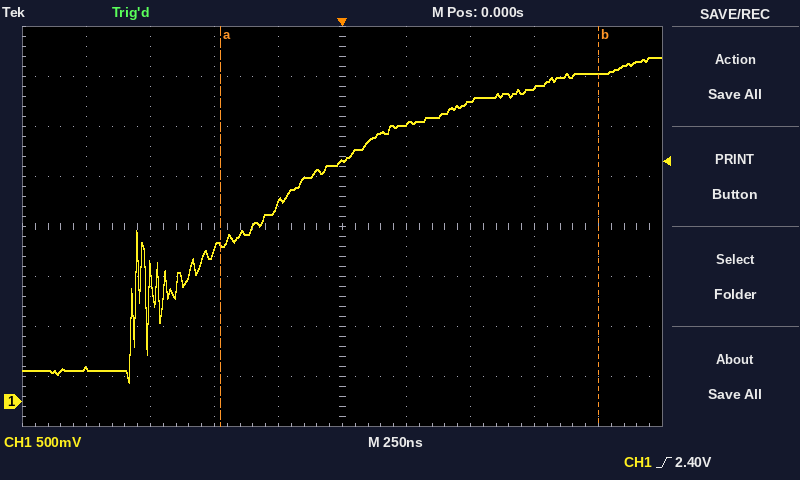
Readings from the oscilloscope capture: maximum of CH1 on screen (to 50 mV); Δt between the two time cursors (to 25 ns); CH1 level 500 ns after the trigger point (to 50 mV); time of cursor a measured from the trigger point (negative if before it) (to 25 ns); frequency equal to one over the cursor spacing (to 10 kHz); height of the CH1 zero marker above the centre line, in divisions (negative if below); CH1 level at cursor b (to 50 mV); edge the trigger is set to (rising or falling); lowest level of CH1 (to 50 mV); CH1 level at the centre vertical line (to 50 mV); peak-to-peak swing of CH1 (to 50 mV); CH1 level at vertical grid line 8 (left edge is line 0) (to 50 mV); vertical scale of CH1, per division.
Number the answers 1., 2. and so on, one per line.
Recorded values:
1. 3.45 V
2. 1.475 µs
3. 3.00 V
4. -475 ns
5. 680 kHz
6. -3.5 div
7. 3.30 V
8. rising
9. 200 mV
10. 2.40 V
11. 3.25 V
12. 3.15 V
13. 500 mV
